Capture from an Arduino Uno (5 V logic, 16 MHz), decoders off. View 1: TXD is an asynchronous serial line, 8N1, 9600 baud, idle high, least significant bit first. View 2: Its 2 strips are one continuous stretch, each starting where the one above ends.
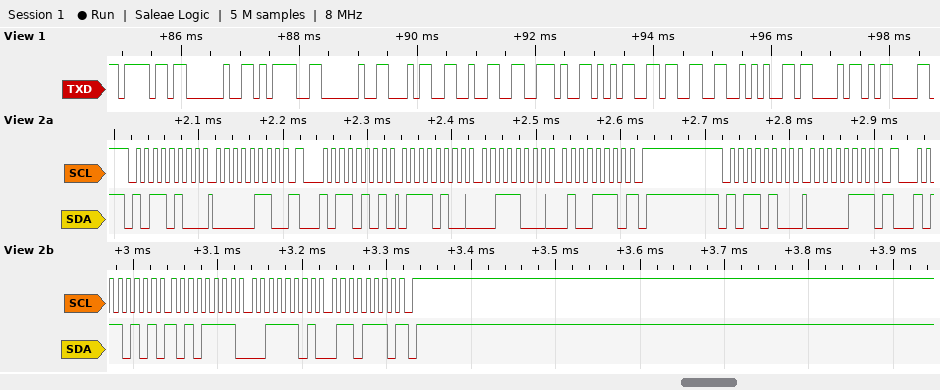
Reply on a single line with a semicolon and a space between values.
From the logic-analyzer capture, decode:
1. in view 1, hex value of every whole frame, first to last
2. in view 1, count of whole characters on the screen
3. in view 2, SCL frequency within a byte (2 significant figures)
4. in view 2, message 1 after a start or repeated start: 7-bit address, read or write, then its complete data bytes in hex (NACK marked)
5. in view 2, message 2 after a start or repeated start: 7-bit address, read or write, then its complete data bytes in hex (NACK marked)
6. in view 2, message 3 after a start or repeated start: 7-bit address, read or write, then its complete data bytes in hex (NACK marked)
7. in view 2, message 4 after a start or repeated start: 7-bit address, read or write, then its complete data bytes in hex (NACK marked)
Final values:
6F 20 3D 20 34 32 2E 35 33 2A 43 0D; 12; 100 kHz; 0x5A write: 06; 0x5A read: 74 38 4E NACK; 0x5A write: 07; 0x5A read: AF 3D 6E NACK
